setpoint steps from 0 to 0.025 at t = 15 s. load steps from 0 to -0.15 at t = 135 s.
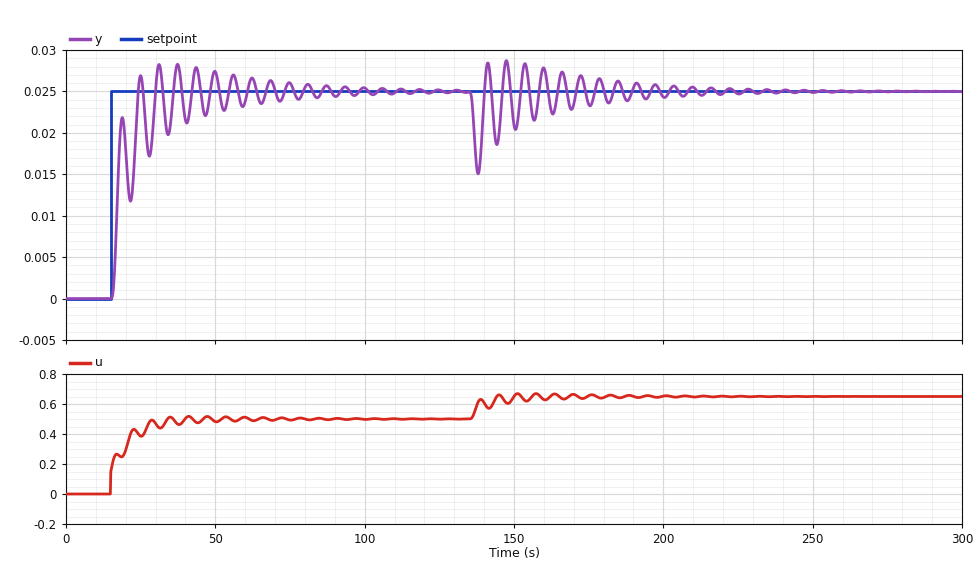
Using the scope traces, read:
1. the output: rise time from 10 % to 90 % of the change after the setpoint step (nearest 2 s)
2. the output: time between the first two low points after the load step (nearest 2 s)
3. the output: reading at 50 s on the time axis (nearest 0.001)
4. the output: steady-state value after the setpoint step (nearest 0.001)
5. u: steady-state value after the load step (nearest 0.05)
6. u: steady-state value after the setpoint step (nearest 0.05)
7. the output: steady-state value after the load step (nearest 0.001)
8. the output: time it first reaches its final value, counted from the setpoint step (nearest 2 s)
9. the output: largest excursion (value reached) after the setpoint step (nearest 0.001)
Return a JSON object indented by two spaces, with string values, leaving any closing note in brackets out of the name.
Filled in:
{
  "the output: rise time from 10 % to 90 % of the change after the setpoint step": "8 s",
  "the output: time between the first two low points after the load step": "6 s",
  "the output: reading at 50 s on the time axis": "0.027",
  "the output: steady-state value after the setpoint step": "0.025",
  "u: steady-state value after the load step": "0.65",
  "u: steady-state value after the setpoint step": "0.50",
  "the output: steady-state value after the load step": "0.025",
  "the output: time it first reaches its final value, counted from the setpoint step": "10 s",
  "the output: largest excursion (value reached) after the setpoint step": "0.028"
}
